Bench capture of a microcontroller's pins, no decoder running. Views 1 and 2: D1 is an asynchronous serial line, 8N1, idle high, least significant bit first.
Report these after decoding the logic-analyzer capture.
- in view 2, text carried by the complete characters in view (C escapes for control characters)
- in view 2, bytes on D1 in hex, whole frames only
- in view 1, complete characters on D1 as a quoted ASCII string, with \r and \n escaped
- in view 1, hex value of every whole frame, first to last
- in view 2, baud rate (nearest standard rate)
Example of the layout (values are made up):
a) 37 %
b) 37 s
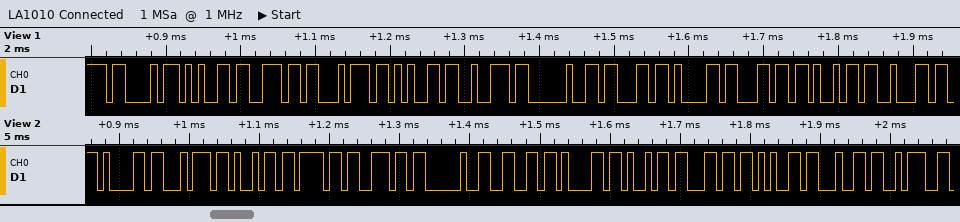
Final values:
a) "ation failed:"
b) 61 74 69 6F 6E 20 66 61 69 6C 65 64 3A
c) "Center calib"
d) 43 65 6E 74 65 72 20 63 61 6C 69 62
e) 115200 baud
